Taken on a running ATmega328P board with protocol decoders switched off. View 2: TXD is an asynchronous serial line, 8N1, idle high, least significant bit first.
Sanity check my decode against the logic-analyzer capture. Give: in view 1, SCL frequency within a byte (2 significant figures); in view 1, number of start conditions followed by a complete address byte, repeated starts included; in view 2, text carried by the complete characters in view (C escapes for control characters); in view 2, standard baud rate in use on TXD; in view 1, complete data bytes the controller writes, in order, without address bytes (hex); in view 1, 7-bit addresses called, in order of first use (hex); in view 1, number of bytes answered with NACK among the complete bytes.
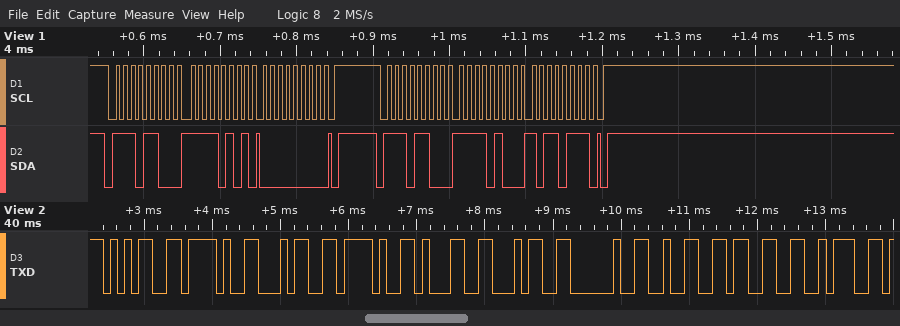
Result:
100 kHz
2
"5/4/14 23:"
9600 baud
F5 00 F4 B7
0x76
0
